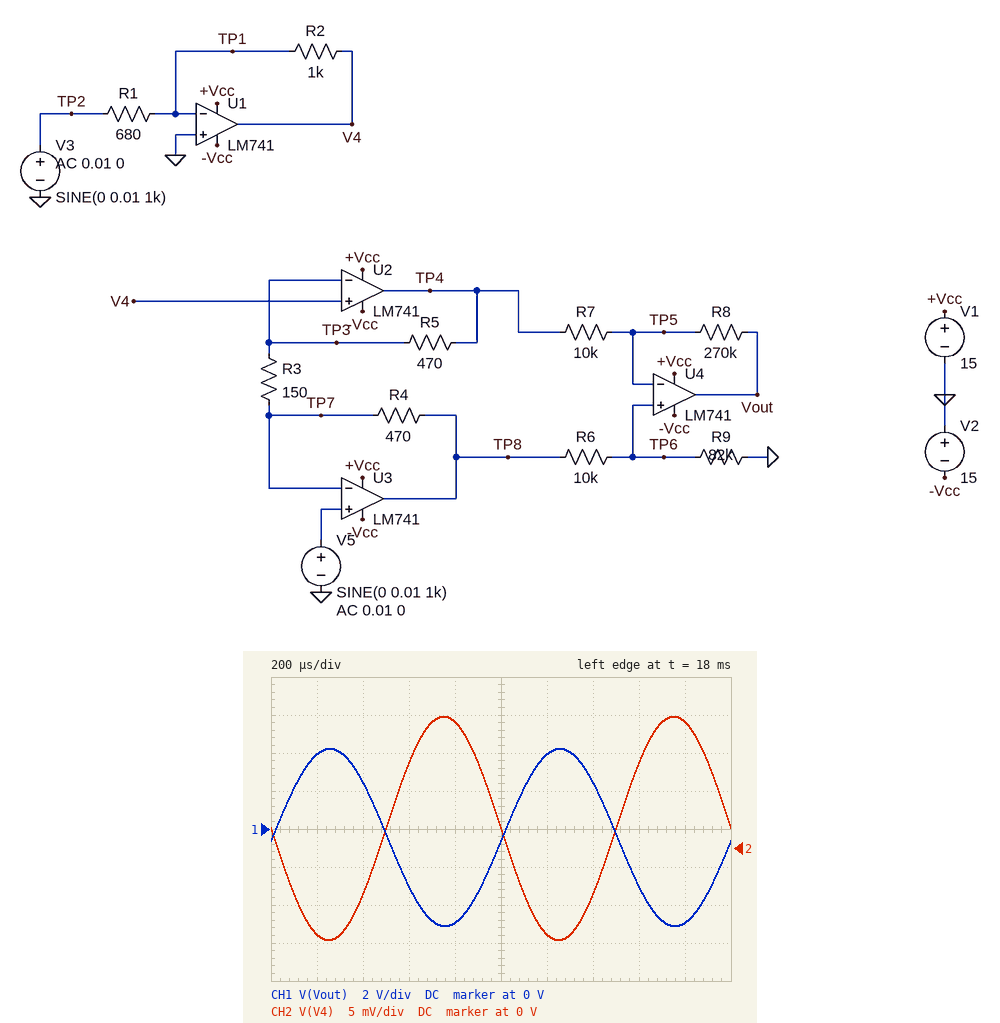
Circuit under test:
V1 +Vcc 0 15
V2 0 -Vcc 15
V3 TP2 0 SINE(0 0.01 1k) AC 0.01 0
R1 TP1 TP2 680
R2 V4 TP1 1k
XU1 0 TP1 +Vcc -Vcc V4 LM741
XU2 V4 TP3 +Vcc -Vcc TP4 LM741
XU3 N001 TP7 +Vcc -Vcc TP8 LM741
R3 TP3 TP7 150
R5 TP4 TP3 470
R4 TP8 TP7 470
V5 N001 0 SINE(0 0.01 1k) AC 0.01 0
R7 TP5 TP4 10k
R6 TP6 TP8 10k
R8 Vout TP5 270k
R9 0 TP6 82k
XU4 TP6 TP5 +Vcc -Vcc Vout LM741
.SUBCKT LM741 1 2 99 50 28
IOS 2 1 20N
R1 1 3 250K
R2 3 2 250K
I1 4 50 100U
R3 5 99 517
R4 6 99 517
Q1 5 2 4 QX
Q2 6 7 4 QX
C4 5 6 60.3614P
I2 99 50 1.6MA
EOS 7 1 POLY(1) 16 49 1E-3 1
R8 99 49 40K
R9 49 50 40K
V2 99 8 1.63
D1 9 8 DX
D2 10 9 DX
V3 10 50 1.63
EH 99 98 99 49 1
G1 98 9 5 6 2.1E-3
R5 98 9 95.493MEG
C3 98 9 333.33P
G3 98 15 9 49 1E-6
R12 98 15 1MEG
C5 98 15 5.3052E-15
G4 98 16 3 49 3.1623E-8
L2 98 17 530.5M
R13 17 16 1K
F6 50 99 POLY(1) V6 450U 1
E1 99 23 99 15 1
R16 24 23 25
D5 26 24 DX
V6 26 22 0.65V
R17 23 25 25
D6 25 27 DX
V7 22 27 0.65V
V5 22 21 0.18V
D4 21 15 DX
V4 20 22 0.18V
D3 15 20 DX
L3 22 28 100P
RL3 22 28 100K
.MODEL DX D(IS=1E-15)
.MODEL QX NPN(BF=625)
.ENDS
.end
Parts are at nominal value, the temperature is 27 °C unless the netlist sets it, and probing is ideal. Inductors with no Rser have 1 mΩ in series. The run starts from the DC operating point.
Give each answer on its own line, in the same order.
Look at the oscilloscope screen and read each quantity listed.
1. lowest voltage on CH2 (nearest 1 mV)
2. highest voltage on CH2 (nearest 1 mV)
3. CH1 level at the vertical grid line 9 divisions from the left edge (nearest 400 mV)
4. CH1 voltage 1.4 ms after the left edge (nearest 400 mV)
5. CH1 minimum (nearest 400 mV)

-12 mV
17 mV
-4.8 V
2.4 V
-5.2 V
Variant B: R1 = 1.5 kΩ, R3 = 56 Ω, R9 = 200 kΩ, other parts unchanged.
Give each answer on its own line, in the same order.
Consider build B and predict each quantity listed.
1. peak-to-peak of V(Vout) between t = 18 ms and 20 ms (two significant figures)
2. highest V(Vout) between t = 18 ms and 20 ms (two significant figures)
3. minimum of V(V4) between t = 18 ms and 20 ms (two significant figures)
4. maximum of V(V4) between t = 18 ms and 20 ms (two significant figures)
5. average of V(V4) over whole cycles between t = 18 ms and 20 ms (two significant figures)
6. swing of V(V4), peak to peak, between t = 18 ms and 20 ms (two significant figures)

16 V
7.1 V
-4.9 mV
8.4 mV
1.8 mV
13 mV
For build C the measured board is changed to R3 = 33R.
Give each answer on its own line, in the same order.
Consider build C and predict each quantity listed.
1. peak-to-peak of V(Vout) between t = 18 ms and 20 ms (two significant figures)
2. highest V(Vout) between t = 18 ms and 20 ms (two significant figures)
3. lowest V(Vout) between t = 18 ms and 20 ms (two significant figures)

28 V
14 V
-14 V
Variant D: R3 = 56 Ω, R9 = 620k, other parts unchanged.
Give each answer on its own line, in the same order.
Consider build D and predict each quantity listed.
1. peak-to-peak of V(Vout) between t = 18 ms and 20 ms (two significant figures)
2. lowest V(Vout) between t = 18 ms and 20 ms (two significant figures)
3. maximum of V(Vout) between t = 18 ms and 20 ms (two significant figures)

24 V
-13 V
11 V
